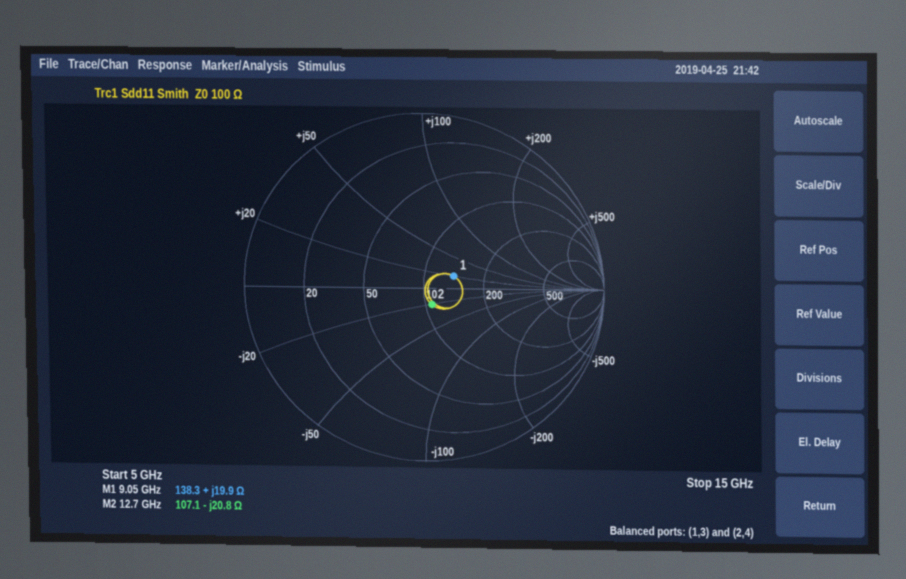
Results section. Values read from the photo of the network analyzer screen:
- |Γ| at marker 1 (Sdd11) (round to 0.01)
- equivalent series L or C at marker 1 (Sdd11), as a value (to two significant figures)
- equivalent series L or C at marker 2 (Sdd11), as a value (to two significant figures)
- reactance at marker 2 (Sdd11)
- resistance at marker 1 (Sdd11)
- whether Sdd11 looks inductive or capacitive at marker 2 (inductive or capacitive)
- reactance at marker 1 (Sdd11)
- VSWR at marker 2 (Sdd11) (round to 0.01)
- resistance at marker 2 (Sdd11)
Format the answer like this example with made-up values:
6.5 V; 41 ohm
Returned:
0.18; 350 pH; 600 fF; -20.8 Ω; 138.3 Ω; capacitive; +19.9 Ω; 1.24; 107.1 Ω
